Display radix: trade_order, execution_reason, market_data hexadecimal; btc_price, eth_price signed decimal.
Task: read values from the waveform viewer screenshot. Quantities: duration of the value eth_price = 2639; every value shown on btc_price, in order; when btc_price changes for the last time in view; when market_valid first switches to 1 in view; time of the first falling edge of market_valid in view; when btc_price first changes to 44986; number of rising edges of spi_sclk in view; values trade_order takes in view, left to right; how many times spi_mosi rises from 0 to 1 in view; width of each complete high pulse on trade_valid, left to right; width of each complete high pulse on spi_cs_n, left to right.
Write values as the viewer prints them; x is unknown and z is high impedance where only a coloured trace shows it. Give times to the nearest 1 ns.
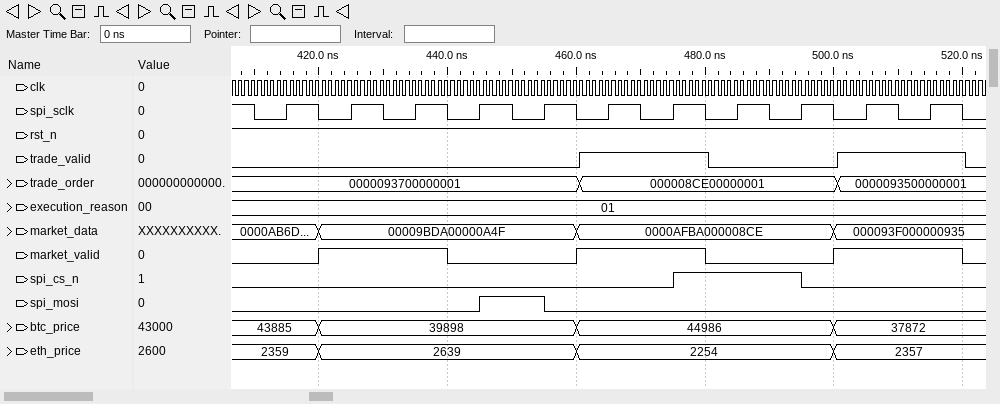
40 ns
43885, 39898, 44986, 37872
500 ns
420 ns
440 ns
460 ns
11
0000093700000001, 000008CE00000001, 0000093500000001
1
20 ns, 20 ns
20 ns
